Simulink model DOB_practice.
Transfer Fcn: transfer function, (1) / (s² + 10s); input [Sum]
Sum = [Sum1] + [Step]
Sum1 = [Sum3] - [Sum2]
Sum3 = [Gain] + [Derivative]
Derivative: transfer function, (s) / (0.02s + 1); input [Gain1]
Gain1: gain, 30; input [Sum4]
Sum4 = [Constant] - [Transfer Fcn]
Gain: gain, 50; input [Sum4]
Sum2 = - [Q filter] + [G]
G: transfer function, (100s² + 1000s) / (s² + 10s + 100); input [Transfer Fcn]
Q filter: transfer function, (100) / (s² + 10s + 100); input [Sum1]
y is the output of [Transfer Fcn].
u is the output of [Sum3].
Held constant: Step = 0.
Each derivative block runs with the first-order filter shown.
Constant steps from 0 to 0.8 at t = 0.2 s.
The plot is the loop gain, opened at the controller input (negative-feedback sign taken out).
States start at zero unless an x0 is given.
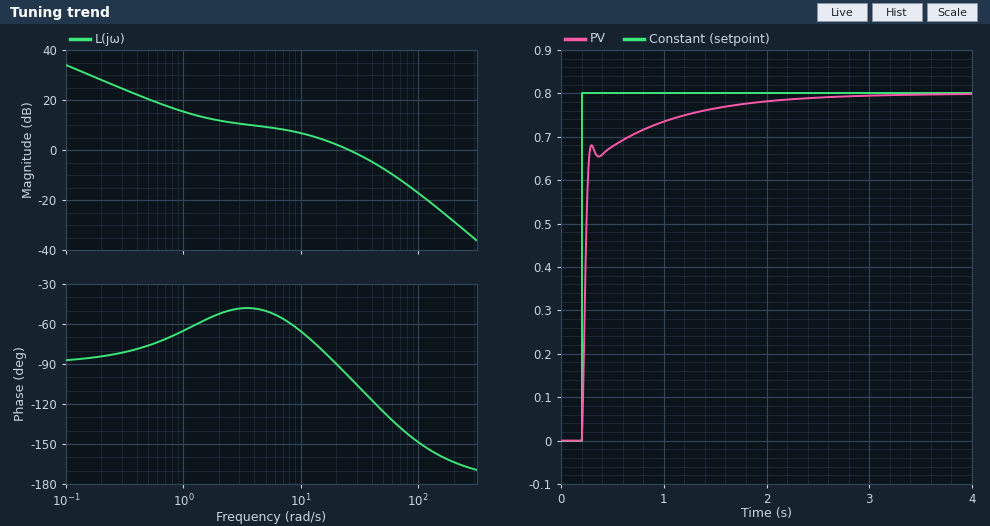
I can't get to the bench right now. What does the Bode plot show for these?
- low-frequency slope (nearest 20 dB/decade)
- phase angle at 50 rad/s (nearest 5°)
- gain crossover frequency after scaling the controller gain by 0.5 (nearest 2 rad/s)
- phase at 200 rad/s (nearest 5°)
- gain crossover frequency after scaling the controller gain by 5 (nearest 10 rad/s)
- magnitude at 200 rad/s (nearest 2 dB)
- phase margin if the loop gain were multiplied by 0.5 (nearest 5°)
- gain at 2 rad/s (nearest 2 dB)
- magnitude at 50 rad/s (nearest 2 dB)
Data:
-20 dB/decade
-125°
12 rad/s
-165°
80 rad/s
-28 dB
110°
12 dB
-8 dB
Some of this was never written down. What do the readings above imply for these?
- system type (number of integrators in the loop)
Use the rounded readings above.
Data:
1
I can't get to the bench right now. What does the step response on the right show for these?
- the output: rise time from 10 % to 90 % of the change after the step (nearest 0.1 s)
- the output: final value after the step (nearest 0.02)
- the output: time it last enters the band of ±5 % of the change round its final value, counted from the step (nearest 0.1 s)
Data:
0.6 s
0.80
1.2 s
